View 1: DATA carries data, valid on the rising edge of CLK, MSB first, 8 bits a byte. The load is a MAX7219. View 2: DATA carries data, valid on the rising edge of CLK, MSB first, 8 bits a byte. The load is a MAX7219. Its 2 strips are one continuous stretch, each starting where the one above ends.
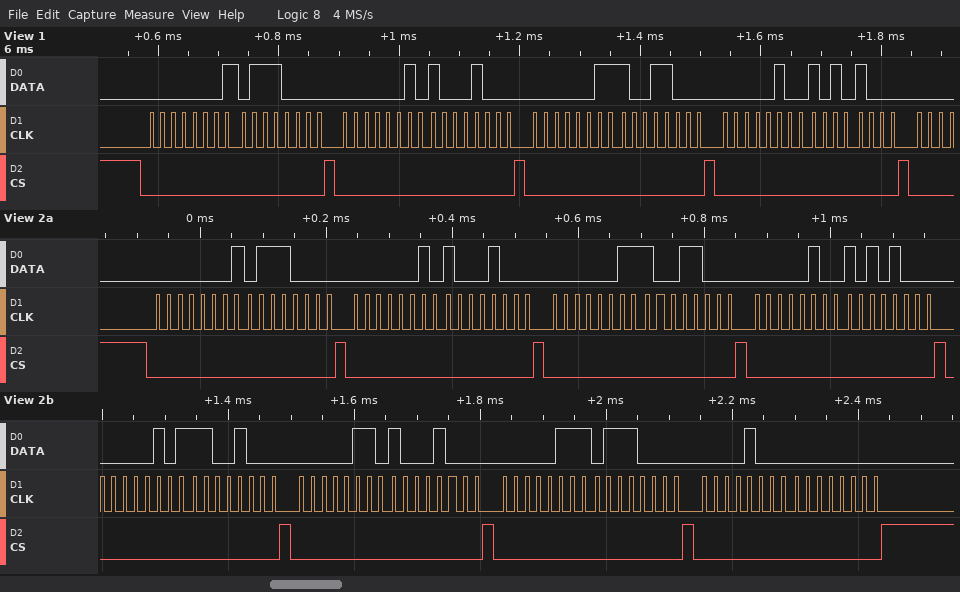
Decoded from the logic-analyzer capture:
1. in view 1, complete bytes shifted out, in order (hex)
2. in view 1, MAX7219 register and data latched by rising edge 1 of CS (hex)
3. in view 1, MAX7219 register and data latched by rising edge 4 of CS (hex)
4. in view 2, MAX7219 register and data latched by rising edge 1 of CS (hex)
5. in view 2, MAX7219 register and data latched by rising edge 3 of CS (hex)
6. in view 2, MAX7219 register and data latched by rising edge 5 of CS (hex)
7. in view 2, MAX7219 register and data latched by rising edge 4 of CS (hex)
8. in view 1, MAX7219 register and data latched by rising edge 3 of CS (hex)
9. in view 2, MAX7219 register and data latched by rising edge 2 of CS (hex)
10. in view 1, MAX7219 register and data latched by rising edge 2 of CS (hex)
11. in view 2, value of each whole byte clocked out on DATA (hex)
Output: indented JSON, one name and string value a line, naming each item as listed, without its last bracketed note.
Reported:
{
  "in view 1, complete bytes shifted out, in order": "01 70 02 88 03 98 04 A8",
  "in view 1, MAX7219 register and data latched by rising edge 1 of CS": "register 0x1, data 0x70",
  "in view 1, MAX7219 register and data latched by rising edge 4 of CS": "register 0x4, data 0xA8",
  "in view 2, MAX7219 register and data latched by rising edge 1 of CS": "register 0x1, data 0x70",
  "in view 2, MAX7219 register and data latched by rising edge 3 of CS": "register 0x3, data 0x98",
  "in view 2, MAX7219 register and data latched by rising edge 5 of CS": "register 0x5, data 0xC8",
  "in view 2, MAX7219 register and data latched by rising edge 4 of CS": "register 0x4, data 0xA8",
  "in view 1, MAX7219 register and data latched by rising edge 3 of CS": "register 0x3, data 0x98",
  "in view 2, MAX7219 register and data latched by rising edge 2 of CS": "register 0x2, data 0x88",
  "in view 1, MAX7219 register and data latched by rising edge 2 of CS": "register 0x2, data 0x88",
  "in view 2, value of each whole byte clocked out on DATA": "0x01 0x70 0x02 0x88 0x03 0x98 0x04 0xA8 0x05 0xC8 0x06 0x88 0x07 0x70 0x08 0x00"
}
